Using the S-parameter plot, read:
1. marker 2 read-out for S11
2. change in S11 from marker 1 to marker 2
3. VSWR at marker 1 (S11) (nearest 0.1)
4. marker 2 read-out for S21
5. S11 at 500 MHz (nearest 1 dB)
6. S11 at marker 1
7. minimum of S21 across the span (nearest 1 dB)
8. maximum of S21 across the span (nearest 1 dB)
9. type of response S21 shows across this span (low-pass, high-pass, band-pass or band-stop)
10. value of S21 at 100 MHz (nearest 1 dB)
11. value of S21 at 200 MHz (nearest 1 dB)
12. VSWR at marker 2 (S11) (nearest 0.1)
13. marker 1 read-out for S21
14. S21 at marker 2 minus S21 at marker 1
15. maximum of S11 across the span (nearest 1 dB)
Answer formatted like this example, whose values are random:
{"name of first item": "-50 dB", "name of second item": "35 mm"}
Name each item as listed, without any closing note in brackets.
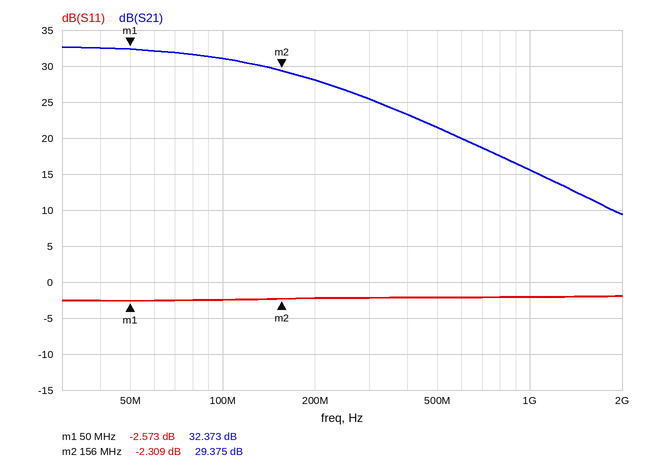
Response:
{"marker 2 read-out for S11": "-2.309 dB", "change in S11 from marker 1 to marker 2": "0.264 dB", "VSWR at marker 1 (S11)": "6.8", "marker 2 read-out for S21": "29.375 dB", "S11 at 500 MHz": "-2 dB", "S11 at marker 1": "-2.573 dB", "minimum of S21 across the span": "9 dB", "maximum of S21 across the span": "33 dB", "type of response S21 shows across this span": "low-pass", "value of S21 at 100 MHz": "31 dB", "value of S21 at 200 MHz": "28 dB", "VSWR at marker 2 (S11)": "7.6", "marker 1 read-out for S21": "32.373 dB", "S21 at marker 2 minus S21 at marker 1": "-2.998 dB", "maximum of S11 across the span": "-2 dB"}
